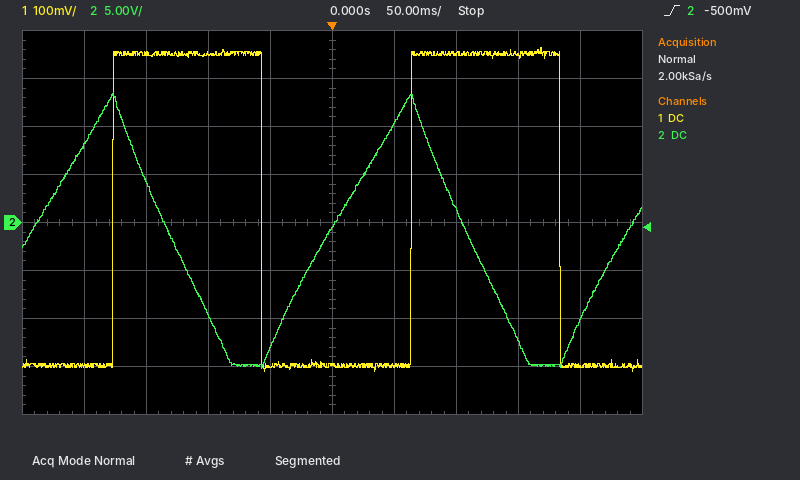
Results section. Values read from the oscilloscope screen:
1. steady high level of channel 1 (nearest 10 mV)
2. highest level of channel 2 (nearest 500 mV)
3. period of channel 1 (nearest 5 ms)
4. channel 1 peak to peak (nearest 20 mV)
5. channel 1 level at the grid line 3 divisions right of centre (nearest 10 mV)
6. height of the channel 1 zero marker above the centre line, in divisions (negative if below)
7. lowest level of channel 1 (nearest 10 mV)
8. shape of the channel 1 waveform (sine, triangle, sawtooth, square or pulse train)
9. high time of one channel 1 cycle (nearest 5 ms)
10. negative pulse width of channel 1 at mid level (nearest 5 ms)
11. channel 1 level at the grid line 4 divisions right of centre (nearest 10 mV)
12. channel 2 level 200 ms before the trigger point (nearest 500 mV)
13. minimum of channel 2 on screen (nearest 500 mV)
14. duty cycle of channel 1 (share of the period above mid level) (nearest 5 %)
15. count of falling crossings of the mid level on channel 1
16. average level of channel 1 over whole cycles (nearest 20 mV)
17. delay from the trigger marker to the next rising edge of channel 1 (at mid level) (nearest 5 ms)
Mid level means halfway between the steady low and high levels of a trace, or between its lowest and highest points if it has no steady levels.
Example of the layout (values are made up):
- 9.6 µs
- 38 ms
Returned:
- 350 mV
- 13.5 V
- 240 ms
- 680 mV
- 350 mV
- 0.0 div
- -310 mV
- square
- 120 ms
- 120 ms
- -300 mV
- 8.0 V
- -15.0 V
- 50 %
- 2
- 20 mV
- 65 ms
